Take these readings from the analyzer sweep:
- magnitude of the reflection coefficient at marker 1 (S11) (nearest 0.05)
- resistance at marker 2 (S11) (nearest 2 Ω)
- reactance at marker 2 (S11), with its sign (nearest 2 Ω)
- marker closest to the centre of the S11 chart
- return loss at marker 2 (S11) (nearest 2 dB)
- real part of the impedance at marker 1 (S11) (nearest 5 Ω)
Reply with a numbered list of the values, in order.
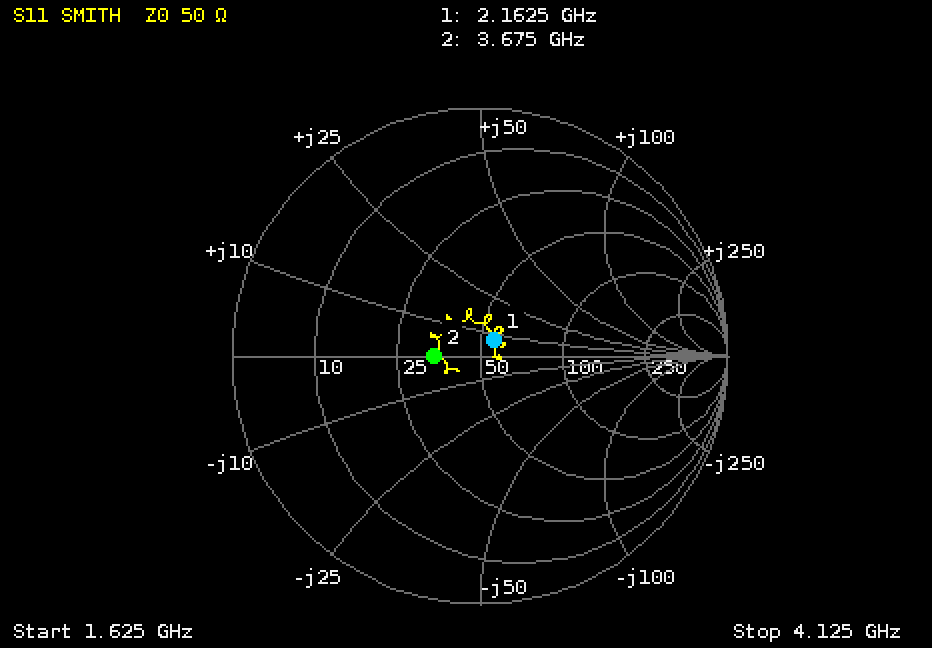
1. 0.10
2. 34 Ω
3. 0 Ω
4. marker 1
5. 14 dB
6. 55 Ω
